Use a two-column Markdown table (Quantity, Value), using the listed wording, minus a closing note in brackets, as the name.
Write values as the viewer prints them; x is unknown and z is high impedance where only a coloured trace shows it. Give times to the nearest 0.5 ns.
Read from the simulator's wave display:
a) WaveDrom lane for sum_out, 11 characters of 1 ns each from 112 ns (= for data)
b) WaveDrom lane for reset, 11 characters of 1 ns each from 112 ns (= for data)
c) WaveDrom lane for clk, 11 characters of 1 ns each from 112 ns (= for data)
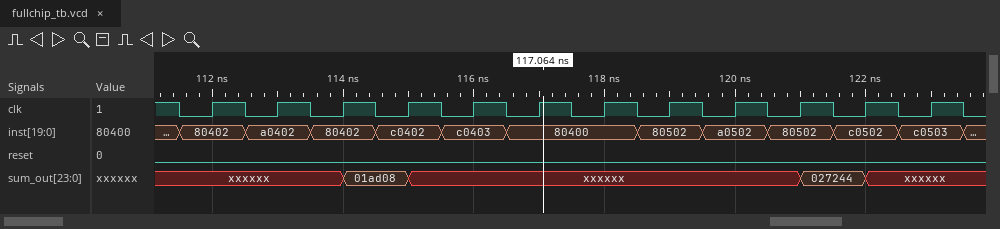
| Quantity | Value |
|---|---|
| WaveDrom lane for sum_out, 11 characters of 1 ns each from 112 ns | {name: 'sum_out', wave: 'x.=x.....=x', data: '01ad08 027244'} |
| WaveDrom lane for reset, 11 characters of 1 ns each from 112 ns | {name: 'reset', wave: '0..........'} |
| WaveDrom lane for clk, 11 characters of 1 ns each from 112 ns | {name: 'clk', wave: 'p..........'} |
